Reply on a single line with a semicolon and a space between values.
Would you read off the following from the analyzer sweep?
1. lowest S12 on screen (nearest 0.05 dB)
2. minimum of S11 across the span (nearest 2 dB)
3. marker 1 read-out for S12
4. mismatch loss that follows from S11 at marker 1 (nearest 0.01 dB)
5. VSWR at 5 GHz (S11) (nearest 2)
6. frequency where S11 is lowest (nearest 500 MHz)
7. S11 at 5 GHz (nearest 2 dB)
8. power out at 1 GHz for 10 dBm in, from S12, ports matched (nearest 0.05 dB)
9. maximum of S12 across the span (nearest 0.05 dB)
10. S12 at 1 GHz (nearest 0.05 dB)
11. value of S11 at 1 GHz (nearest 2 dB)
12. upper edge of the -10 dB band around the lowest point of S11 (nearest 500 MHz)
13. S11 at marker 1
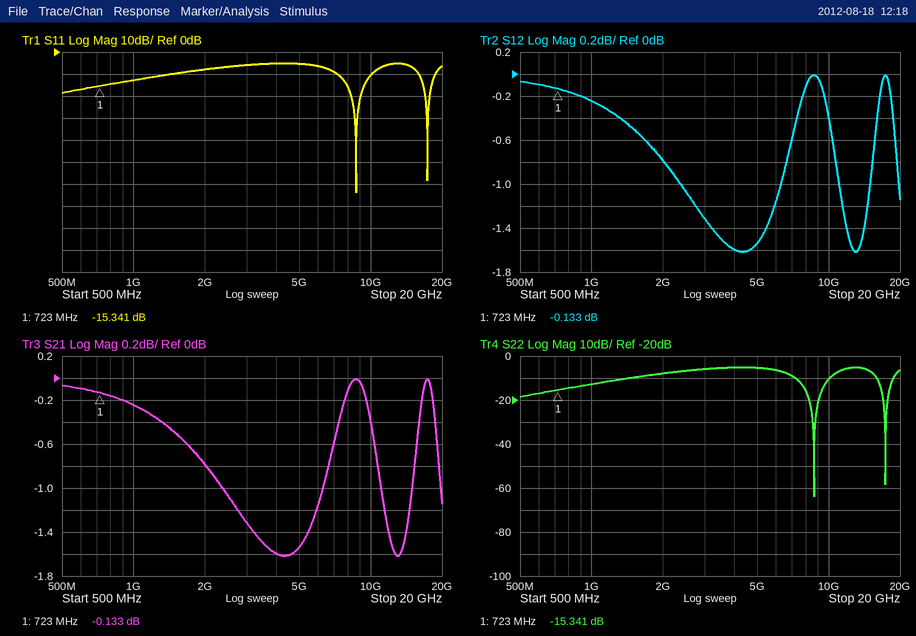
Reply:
-1.60 dB; -64 dB; -0.133 dB; 0.13 dB; 4; 8.5 GHz; -6 dB; 9.75 dBm; 0.00 dB; -0.25 dB; -12 dB; 10.0 GHz; -15.341 dB
